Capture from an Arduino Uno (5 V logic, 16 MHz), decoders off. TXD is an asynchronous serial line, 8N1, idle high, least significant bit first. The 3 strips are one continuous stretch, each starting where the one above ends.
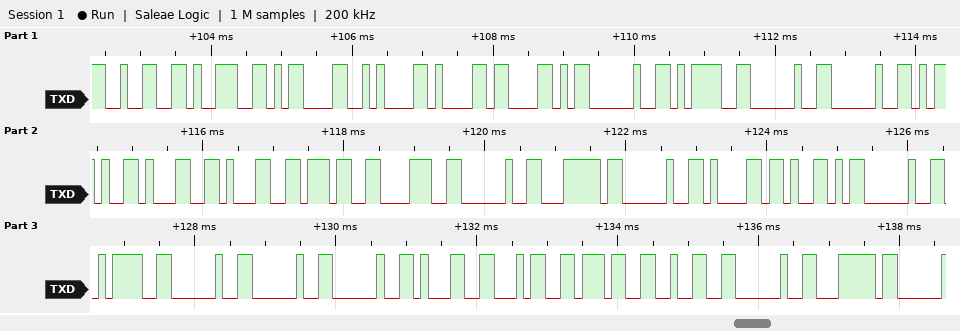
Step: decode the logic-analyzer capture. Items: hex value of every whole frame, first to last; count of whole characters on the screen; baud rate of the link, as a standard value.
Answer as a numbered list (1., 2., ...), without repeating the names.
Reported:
1. 32 39 0D 0A 61 58 20 3D 20 20 2D 31 31 37 38 20 7C 20 61 59 20 3D 20 20 20 31 34 37 32 20 7C
2. 31
3. 9600 baud
